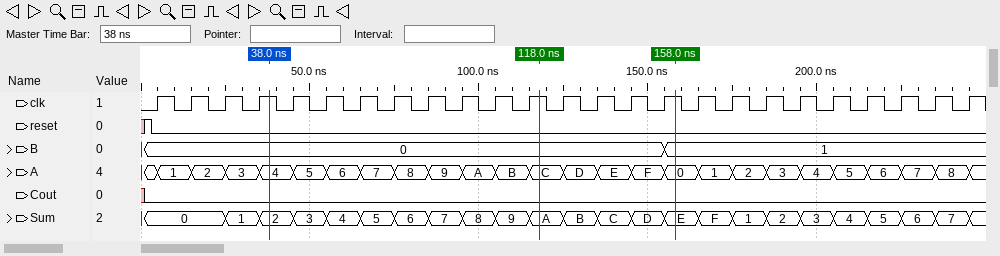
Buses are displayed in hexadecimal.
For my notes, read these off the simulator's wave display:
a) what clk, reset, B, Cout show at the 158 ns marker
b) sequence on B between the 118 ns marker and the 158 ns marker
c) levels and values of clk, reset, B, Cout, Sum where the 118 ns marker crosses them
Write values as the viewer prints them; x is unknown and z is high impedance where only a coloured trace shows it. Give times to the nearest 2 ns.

clk=1, reset=0, B=1, Cout=0
0, 1
clk=1, reset=0, B=0, Cout=0, Sum=A
